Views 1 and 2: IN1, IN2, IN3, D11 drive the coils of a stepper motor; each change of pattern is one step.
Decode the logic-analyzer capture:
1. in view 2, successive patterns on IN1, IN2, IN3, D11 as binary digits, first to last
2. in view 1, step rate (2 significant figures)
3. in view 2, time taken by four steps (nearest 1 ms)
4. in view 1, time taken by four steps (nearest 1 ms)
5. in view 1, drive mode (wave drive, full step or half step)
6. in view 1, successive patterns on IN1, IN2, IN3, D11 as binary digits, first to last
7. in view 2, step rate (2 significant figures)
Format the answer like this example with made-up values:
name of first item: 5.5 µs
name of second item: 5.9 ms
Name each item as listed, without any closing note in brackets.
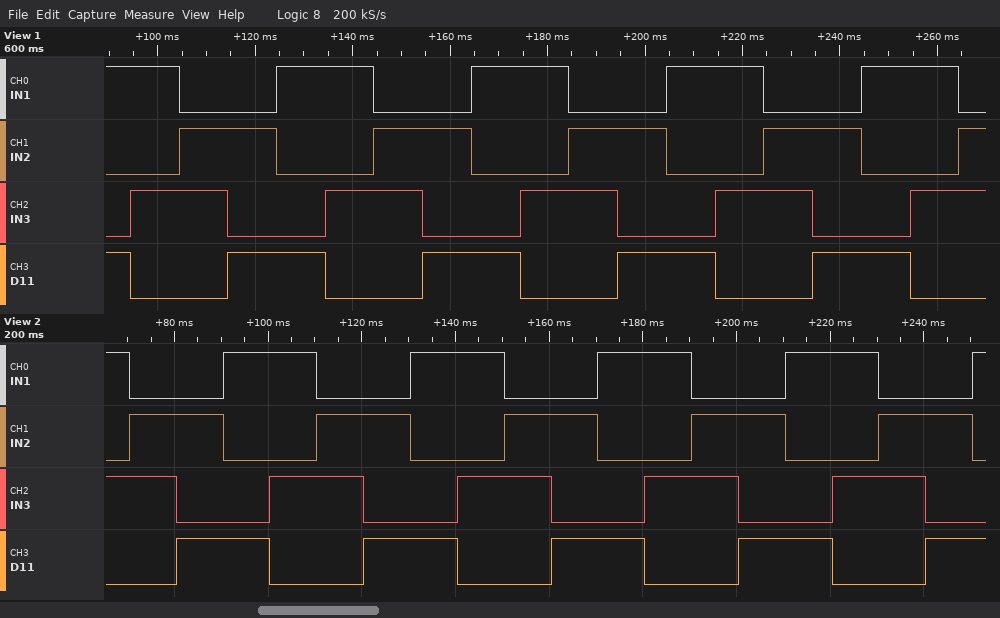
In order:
in view 2, successive patterns on IN1, IN2, IN3, D11 as binary digits, first to last: 1010 0110 0101 1001 1010 0110 0101 1001 1010 0110 0101 1001 1010 0110 0101 1001 1010 0110 0101 1001
in view 1, step rate: 100 steps/s
in view 2, time taken by four steps: 40 ms
in view 1, time taken by four steps: 40 ms
in view 1, drive mode: full step
in view 1, successive patterns on IN1, IN2, IN3, D11 as binary digits, first to last: 1001 1010 0110 0101 1001 1010 0110 0101 1001 1010 0110 0101 1001 1010 0110 0101 1001 1010 0110
in view 2, step rate: 100 steps/s
